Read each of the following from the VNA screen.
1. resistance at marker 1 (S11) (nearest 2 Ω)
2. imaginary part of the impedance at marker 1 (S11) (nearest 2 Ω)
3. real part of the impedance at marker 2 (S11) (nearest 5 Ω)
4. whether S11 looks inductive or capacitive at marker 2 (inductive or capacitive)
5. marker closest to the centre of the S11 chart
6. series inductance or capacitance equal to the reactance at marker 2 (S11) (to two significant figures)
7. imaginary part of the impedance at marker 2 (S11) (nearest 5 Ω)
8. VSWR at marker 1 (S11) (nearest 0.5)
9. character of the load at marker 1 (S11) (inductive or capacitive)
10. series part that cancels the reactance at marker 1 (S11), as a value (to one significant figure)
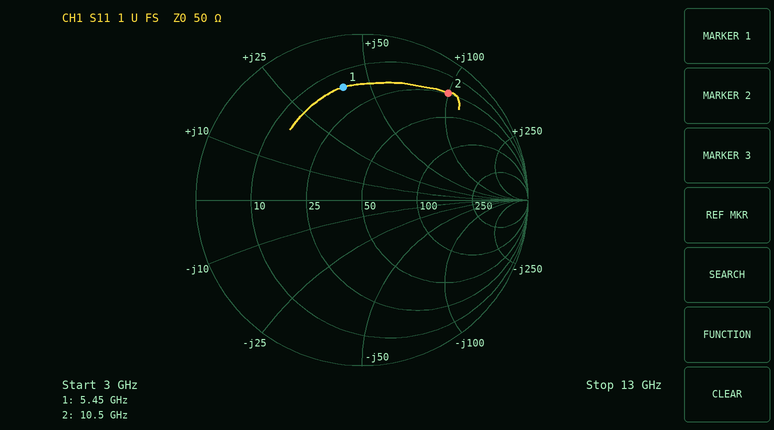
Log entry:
16 Ω
+40 Ω
25 Ω
inductive
marker 1
1.5 nH
+100 Ω
5.5
inductive
700 fF
